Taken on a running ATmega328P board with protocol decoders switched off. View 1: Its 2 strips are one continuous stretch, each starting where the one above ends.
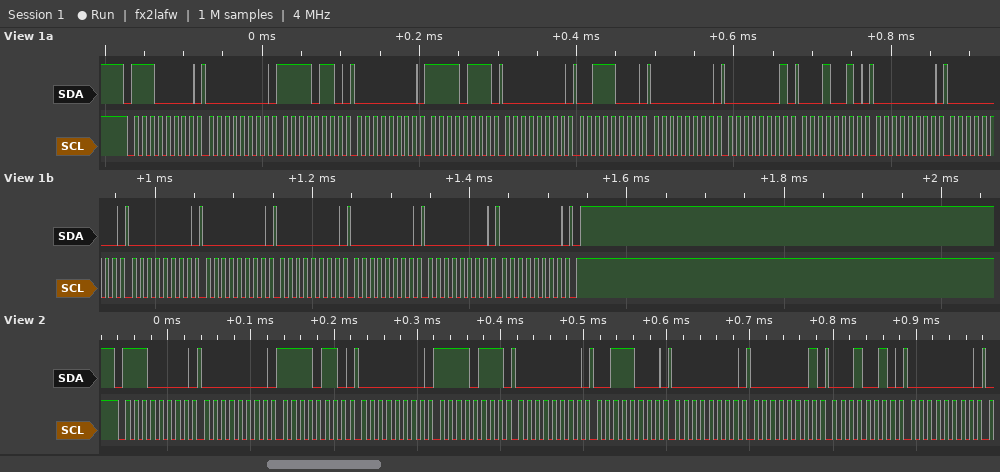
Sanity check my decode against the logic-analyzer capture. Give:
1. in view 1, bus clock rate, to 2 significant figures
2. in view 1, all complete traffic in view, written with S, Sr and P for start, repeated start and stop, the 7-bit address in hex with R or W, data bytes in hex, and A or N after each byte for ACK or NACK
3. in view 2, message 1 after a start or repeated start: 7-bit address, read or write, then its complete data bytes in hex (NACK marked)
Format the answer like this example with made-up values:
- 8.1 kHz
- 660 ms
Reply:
- 100 kHz
- S 70W A 00 A F6 A 00 A F7 A 00 A 38 A 00 A 01 A 12 A 00 A 00 A 00 A 00 A 00 A 00 A 00 A 00 A P
- 0x70 write: 00 F6 00 F7 00 38 00 01 12 00
